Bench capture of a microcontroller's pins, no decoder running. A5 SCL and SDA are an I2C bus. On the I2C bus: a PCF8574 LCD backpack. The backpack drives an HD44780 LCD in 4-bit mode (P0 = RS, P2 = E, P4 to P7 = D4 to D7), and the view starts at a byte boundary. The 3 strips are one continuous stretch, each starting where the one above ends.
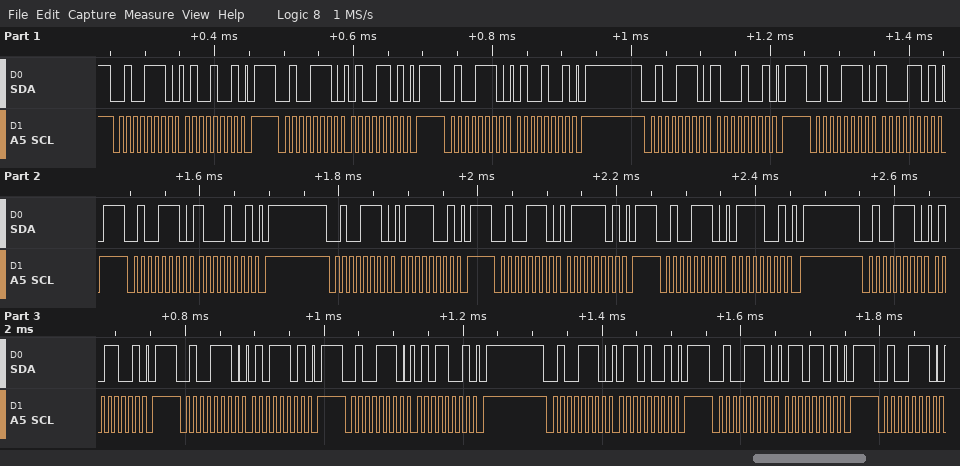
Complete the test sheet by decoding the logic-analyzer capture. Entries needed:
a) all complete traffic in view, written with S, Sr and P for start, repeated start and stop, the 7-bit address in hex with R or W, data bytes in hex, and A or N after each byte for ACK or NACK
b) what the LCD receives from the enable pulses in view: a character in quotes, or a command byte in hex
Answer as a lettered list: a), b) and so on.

a) S 27W A 49 A P S 27W A 4D A P S 27W A 49 A P S 27W A 89 A P S 27W A 8D A P S 27W A 89 A P S 27W A 79 A P S 27W A 7D A P S 27W A 79 A P S 27W A 59 A P S 27W A 5D A P S 27W A 59 A P S 27W A 69 A P S 27W A 6D A P S 27W A
b) 'H' 'u'
